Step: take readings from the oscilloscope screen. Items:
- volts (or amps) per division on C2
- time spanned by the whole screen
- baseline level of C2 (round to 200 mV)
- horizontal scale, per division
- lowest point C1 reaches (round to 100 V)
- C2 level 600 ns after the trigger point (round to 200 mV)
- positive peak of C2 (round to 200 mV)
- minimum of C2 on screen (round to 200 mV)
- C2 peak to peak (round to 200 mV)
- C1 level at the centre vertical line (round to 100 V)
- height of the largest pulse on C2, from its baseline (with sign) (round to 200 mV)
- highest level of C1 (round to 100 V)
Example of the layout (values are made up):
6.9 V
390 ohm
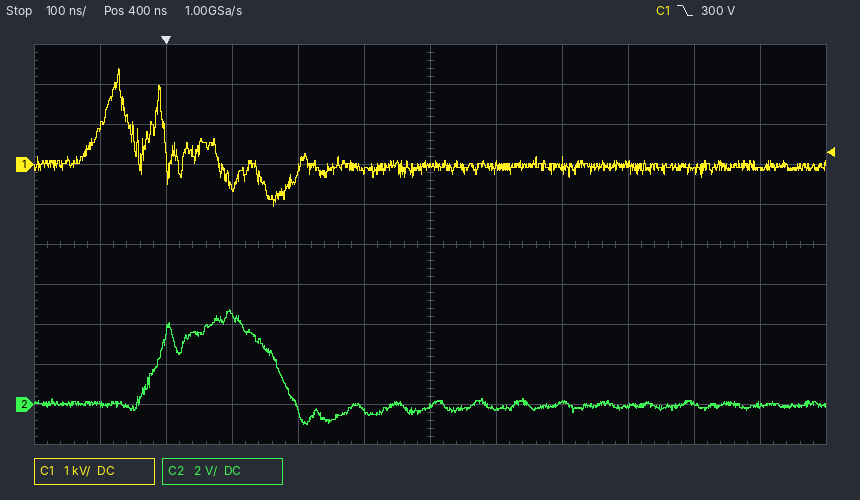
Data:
2 V
1.2 µs
0.0 V
100 ns
-1.0 kV
200 mV
4.8 V
-1.0 V
5.8 V
0.0 kV
+4.8 V
2.4 kV
